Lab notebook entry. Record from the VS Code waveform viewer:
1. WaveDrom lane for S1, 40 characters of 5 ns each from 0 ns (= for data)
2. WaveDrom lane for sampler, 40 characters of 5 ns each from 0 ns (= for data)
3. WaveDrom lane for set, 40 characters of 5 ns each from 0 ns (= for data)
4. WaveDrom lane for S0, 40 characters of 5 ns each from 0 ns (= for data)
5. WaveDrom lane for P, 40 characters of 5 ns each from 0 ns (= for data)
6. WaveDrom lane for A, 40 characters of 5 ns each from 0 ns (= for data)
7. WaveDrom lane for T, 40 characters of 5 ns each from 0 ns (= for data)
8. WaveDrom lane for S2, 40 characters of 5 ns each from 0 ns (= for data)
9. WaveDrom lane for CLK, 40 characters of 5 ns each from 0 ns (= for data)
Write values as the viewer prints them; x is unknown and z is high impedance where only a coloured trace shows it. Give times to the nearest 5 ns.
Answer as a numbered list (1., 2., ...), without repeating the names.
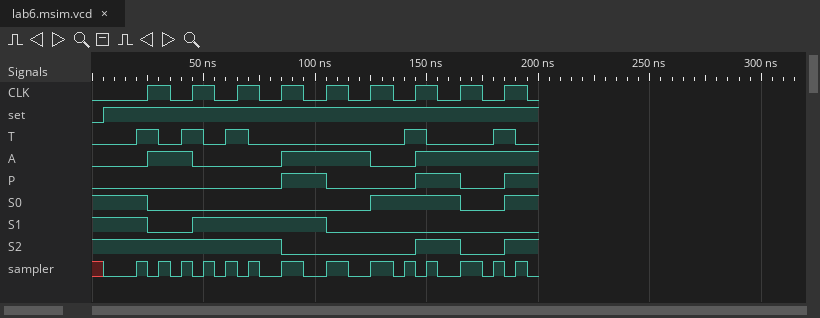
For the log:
1. {name: 'S1', wave: '1....0...1...........0..................'}
2. {name: 'sampler', wave: 'x0..101010101010.1.0.1.0.1.01010.1.01010'}
3. {name: 'set', wave: '01......................................'}
4. {name: 'S0', wave: '1....0...................1.......0...1..'}
5. {name: 'P', wave: '0................1...0.......1...0...1..'}
6. {name: 'A', wave: '0....1...0.......1.......0...1..........'}
7. {name: 'T', wave: '0...1.0.1.0.1.0.............1.0.....1.0.'}
8. {name: 'S2', wave: '1................0...........1...0...1..'}
9. {name: 'CLK', wave: '0....1.0.1.0.1.0.1.0.1.0.1.0.1.0.1.0.1.0'}
